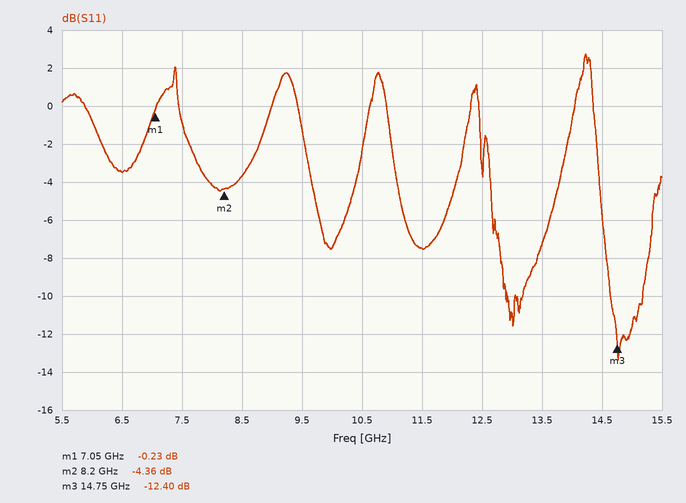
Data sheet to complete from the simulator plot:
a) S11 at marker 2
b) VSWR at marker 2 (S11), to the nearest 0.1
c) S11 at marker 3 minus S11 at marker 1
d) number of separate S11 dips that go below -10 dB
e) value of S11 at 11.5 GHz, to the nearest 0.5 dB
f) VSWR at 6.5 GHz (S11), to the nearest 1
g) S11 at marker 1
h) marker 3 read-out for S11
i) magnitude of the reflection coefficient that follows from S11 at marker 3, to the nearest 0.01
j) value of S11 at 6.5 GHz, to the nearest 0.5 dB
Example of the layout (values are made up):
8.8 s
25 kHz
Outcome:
-4.36 dB
4.1
-12.17 dB
2
-7.5 dB
5
-0.23 dB
-12.40 dB
0.24
-3.5 dB
